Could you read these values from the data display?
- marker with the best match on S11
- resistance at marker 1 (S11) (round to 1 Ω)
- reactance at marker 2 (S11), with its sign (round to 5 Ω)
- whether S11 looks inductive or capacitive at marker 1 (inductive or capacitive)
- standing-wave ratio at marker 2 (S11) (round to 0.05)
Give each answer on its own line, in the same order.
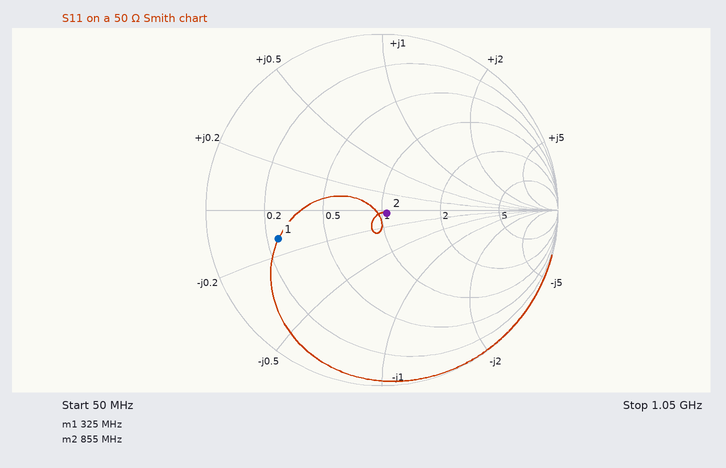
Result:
marker 2
12 Ω
0 Ω
capacitive
1.05
